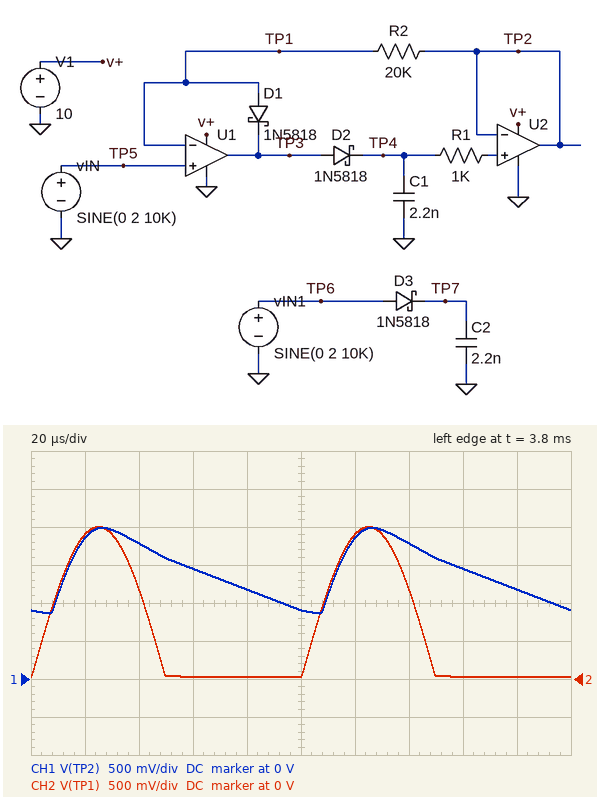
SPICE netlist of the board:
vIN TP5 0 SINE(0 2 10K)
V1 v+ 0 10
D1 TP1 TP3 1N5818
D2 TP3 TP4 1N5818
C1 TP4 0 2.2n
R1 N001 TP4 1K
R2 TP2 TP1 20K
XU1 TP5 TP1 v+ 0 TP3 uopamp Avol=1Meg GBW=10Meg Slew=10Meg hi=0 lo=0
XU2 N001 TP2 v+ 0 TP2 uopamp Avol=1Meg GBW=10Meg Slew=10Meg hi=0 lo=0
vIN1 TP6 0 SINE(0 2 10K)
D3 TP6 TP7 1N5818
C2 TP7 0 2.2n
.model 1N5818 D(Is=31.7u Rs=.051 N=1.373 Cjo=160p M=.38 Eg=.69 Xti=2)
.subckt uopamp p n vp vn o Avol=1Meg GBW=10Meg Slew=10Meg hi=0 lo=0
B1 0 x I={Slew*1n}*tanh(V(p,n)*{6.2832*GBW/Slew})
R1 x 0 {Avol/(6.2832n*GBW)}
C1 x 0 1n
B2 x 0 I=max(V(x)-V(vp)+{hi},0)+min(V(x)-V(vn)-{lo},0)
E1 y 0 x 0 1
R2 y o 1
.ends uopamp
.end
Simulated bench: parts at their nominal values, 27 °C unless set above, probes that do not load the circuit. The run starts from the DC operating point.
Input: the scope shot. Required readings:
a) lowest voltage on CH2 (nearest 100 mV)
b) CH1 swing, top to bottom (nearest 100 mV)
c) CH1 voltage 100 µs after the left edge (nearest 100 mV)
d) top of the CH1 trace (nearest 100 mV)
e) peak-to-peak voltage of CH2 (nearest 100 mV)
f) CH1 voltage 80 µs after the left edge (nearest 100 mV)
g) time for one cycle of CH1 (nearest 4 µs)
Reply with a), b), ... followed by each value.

a) 0 V
b) 1.1 V
c) 900 mV
d) 2.0 V
e) 2.0 V
f) 1.2 V
g) 100 µs
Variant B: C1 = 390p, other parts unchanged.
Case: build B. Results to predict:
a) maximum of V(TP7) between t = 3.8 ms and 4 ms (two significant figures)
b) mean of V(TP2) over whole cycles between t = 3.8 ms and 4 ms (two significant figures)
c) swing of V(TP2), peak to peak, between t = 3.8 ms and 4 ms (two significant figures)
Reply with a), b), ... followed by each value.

a) 2.0 V
b) 670 mV
c) 2.0 V
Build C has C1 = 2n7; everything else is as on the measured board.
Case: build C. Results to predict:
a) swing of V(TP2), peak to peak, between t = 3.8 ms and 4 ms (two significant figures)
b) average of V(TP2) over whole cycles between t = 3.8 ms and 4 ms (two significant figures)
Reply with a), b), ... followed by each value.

a) 940 mV
b) 1.5 V
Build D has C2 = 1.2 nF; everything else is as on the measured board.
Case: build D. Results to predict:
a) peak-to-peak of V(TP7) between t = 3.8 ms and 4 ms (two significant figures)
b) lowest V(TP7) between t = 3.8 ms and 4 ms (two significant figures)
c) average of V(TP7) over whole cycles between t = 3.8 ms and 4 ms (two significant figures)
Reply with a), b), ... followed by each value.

a) 1.9 V
b) 100 mV
c) 1.0 V
